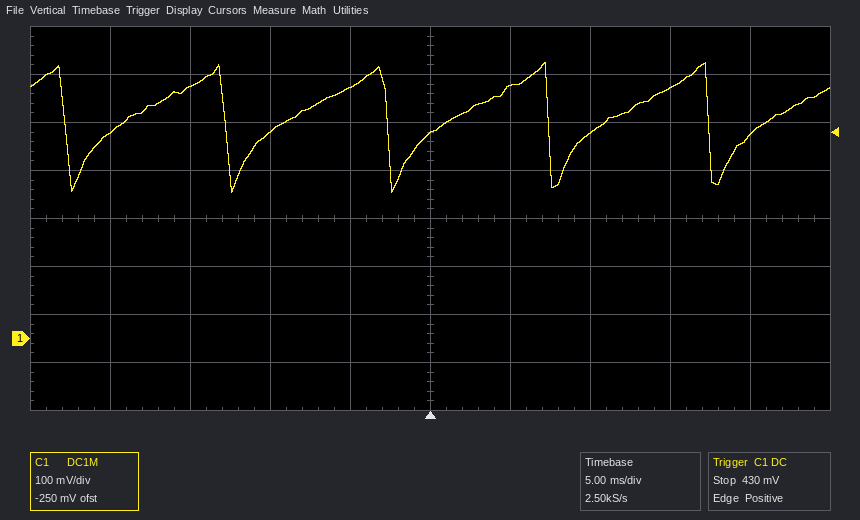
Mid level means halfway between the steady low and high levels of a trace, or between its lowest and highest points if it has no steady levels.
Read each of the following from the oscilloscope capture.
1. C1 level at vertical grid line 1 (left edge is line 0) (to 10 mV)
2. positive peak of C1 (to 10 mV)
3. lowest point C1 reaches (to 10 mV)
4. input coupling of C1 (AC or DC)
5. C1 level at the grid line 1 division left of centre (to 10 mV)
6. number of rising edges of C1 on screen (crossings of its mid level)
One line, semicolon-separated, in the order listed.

430 mV; 580 mV; 300 mV; DC; 520 mV; 5
